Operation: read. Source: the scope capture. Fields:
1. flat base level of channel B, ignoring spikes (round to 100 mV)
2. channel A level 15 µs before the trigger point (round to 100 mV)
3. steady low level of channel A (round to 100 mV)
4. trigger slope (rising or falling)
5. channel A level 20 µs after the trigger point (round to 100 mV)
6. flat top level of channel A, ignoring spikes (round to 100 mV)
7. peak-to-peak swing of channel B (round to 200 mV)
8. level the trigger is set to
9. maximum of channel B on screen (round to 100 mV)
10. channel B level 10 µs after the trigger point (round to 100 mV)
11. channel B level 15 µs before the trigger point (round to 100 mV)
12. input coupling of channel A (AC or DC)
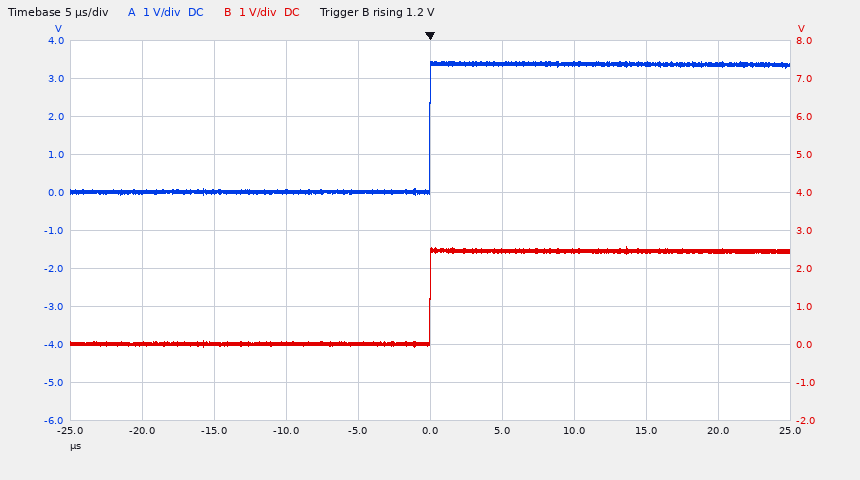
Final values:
0.0 V
0.0 V
0.0 V
rising
3.4 V
3.4 V
2.6 V
1.2 V
2.6 V
2.5 V
0.0 V
DC
